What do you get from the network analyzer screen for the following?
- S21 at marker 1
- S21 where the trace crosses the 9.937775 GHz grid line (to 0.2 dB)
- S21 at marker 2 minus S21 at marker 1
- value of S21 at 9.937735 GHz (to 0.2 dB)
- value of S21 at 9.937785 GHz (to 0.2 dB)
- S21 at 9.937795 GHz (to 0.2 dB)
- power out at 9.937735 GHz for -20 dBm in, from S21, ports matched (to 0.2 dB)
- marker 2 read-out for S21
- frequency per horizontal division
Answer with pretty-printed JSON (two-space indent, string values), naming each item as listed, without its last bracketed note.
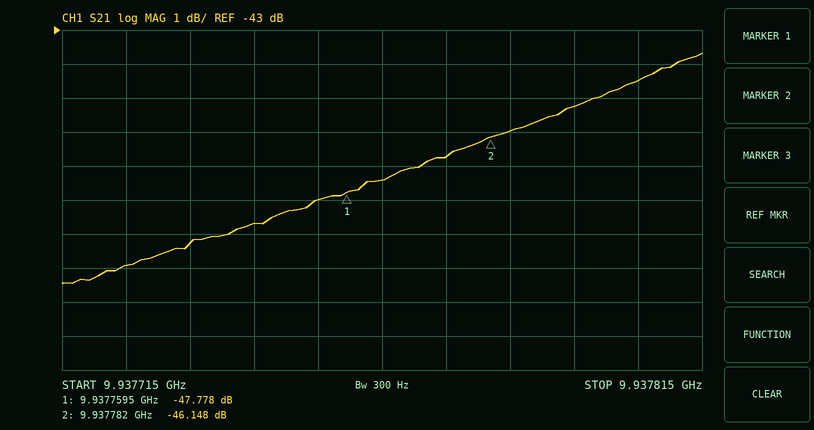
{
  "S21 at marker 1": "-47.778 dB",
  "S21 where the trace crosses the 9.937775 GHz grid line": "-46.8 dB",
  "S21 at marker 2 minus S21 at marker 1": "1.630 dB",
  "value of S21 at 9.937735 GHz": "-49.2 dB",
  "value of S21 at 9.937785 GHz": "-46.0 dB",
  "S21 at 9.937795 GHz": "-45.2 dB",
  "power out at 9.937735 GHz for -20 dBm in, from S21, ports matched": "-69.2 dBm",
  "marker 2 read-out for S21": "-46.148 dB",
  "frequency per horizontal division": "10 kHz"
}
